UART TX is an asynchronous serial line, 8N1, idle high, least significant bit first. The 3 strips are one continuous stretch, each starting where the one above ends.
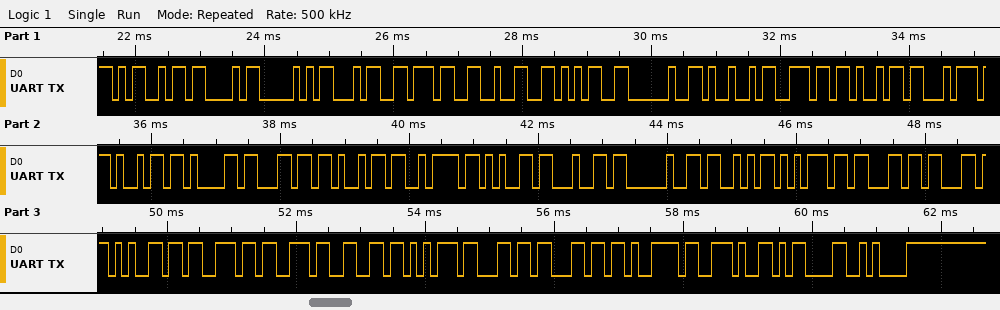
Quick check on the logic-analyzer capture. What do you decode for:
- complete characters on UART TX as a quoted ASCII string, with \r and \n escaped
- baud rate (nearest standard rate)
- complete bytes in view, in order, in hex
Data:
"MCP4725 Initialized Successfully.\r\n"
9600 baud
4D 43 50 34 37 32 35 20 49 6E 69 74 69 61 6C 69 7A 65 64 20 53 75 63 63 65 73 73 66 75 6C 6C 79 2E 0D 0A
